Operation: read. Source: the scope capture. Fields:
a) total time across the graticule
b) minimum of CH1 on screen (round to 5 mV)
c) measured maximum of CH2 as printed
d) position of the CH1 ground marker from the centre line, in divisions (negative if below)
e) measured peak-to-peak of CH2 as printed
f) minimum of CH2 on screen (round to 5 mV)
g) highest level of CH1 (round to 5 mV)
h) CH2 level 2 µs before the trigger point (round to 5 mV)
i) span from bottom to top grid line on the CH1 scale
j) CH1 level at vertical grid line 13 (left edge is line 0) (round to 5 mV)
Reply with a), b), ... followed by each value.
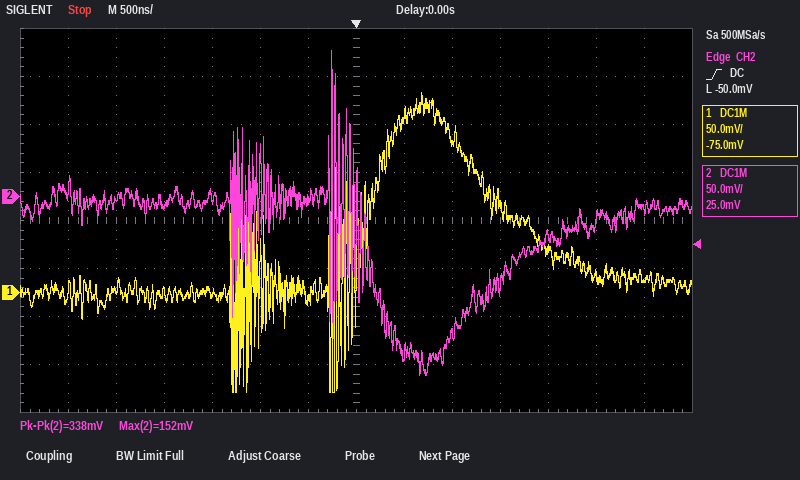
a) 7 µs
b) -105 mV
c) 152 mV
d) -1.5 div
e) 338 mV
f) -185 mV
g) 210 mV
h) -10 mV
i) 400 mV
j) 15 mV
